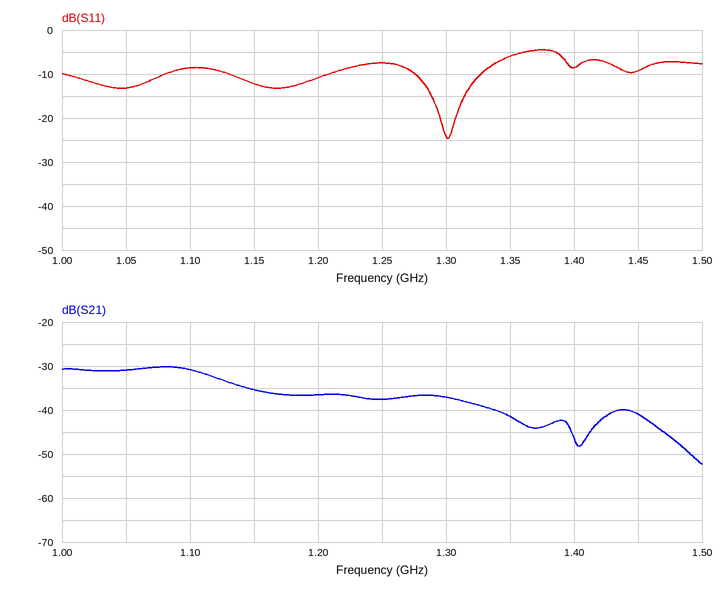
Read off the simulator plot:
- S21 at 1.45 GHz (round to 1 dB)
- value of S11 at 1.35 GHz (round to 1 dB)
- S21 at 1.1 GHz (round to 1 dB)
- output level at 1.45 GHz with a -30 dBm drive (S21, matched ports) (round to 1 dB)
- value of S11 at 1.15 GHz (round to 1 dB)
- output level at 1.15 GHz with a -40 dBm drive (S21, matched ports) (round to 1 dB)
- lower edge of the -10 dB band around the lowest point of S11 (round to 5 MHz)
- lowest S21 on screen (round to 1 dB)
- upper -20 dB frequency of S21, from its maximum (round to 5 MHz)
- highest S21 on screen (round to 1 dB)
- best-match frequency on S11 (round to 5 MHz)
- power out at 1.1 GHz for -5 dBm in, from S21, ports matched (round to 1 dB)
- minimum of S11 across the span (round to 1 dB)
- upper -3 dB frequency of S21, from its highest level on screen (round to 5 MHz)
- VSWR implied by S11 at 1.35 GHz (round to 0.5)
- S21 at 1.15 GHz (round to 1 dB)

-41 dB
-6 dB
-31 dB
-71 dBm
-12 dB
-75 dBm
1.275 GHz
-52 dB
1.490 GHz
-30 dB
1.300 GHz
-36 dBm
-25 dB
1.125 GHz
3.0
-35 dB
